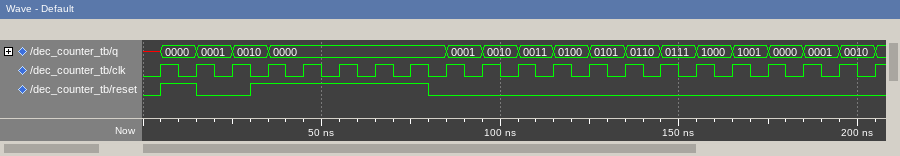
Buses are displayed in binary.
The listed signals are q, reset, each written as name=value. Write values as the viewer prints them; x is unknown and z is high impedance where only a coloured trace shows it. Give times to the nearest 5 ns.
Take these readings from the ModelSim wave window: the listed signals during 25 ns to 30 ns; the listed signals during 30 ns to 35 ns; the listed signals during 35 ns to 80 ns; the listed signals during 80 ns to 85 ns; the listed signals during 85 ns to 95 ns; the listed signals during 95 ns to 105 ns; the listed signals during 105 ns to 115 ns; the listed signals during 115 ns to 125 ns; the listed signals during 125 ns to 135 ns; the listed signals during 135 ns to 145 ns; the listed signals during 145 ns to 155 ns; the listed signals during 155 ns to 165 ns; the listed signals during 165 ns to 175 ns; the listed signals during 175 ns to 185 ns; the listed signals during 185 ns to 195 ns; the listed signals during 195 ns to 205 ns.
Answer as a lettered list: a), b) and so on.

a) q=0010, reset=0
b) q=0010, reset=1
c) q=0000, reset=1
d) q=0000, reset=0
e) q=0001, reset=0
f) q=0010, reset=0
g) q=0011, reset=0
h) q=0100, reset=0
i) q=0101, reset=0
j) q=0110, reset=0
k) q=0111, reset=0
l) q=1000, reset=0
m) q=1001, reset=0
n) q=0000, reset=0
o) q=0001, reset=0
p) q=0010, reset=0
